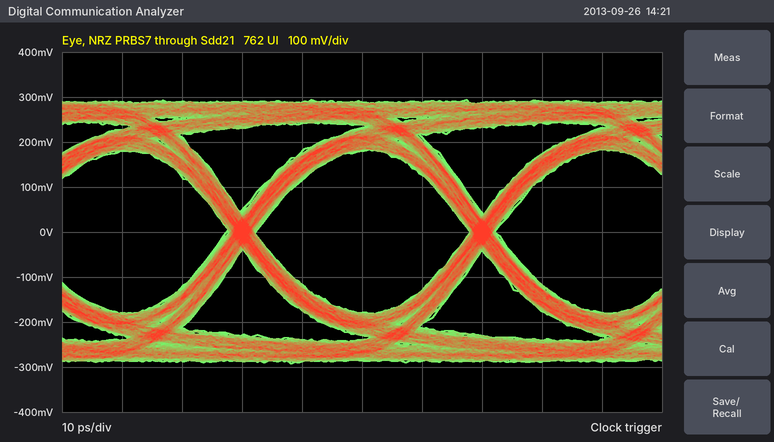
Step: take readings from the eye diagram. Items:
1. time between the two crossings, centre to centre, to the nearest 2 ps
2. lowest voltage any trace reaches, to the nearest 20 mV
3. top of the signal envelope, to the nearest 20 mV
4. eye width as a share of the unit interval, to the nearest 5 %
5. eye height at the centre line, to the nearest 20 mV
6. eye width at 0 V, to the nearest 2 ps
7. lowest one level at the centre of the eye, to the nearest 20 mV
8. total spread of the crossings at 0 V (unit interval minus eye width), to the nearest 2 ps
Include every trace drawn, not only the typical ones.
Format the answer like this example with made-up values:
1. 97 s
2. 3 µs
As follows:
1. 40 ps
2. -300 mV
3. 300 mV
4. 90 %
5. 360 mV
6. 36 ps
7. 180 mV
8. 4 ps
